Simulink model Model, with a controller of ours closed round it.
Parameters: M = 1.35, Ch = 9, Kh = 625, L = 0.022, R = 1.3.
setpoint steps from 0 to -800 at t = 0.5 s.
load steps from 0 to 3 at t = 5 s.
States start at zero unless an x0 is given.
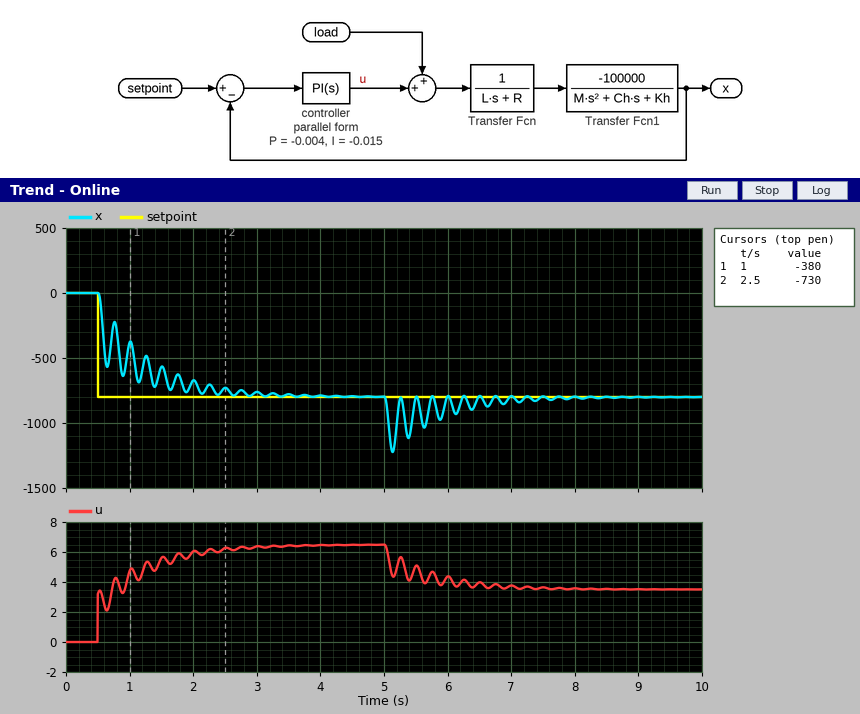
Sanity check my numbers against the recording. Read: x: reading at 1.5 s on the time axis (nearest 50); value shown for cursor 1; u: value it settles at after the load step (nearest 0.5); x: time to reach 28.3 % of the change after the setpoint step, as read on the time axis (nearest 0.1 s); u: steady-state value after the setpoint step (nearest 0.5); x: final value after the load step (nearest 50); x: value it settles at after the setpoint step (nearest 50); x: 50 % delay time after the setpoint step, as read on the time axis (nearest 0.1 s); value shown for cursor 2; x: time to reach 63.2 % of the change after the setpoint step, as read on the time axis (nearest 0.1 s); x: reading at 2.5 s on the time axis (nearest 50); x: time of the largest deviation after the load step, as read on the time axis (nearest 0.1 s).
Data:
-550
-380
3.5
0.6 s
6.5
-800
-800
0.6 s
-730
0.6 s
-750
5.1 s
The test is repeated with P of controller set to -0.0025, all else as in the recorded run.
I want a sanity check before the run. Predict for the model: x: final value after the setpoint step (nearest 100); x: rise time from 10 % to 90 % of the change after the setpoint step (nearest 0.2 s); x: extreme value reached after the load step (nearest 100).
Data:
-800
1.2 s
-1300
